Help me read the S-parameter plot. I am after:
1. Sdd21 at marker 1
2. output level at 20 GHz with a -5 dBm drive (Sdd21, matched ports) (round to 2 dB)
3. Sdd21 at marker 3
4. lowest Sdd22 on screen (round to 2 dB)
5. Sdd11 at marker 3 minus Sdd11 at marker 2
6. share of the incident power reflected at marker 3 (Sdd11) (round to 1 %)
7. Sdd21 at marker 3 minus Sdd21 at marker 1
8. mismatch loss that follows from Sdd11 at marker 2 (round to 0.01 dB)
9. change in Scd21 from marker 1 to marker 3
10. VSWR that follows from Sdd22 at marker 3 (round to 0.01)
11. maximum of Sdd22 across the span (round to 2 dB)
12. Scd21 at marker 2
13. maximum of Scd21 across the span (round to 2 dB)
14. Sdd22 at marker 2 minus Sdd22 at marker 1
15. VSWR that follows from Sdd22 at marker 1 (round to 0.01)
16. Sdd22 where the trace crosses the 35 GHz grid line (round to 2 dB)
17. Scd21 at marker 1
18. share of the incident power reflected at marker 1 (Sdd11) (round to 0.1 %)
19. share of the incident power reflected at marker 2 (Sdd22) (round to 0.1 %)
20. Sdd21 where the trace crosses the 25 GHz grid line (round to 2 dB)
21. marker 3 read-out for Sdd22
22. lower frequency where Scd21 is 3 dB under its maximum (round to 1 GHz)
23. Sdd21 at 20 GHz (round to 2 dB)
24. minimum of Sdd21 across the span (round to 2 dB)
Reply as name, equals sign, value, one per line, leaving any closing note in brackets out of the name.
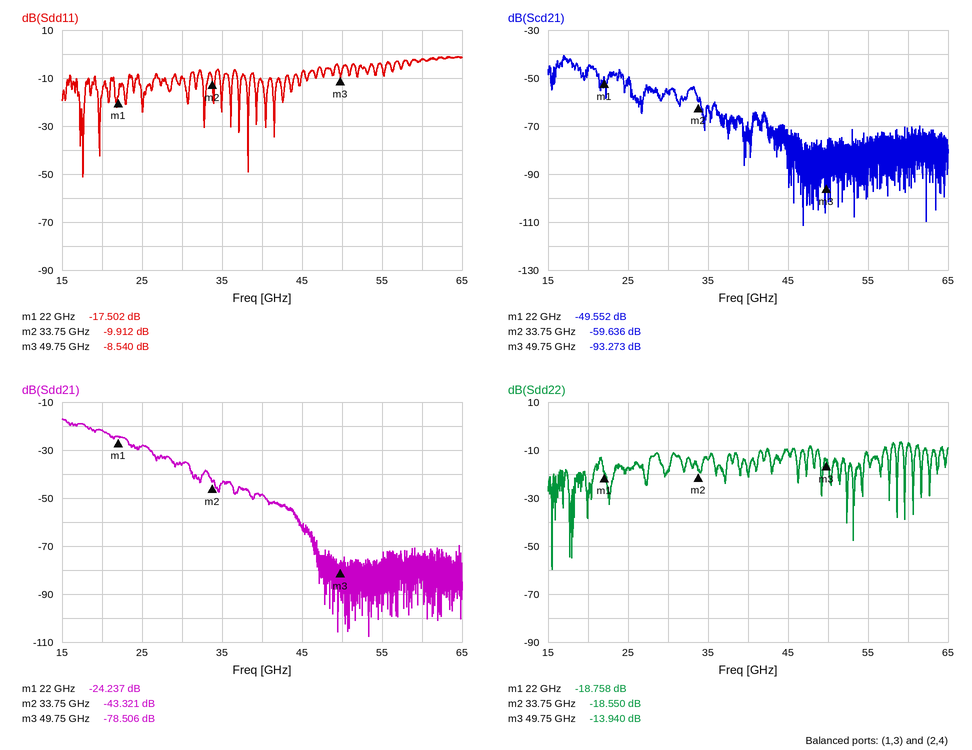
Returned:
Sdd21 at marker 1 = -24.237 dB
output level at 20 GHz with a -5 dBm drive (Sdd21, matched ports) = -26 dBm
Sdd21 at marker 3 = -78.506 dB
lowest Sdd22 on screen = -60 dB
Sdd11 at marker 3 minus Sdd11 at marker 2 = 1.372 dB
share of the incident power reflected at marker 3 (Sdd11) = 14 %
Sdd21 at marker 3 minus Sdd21 at marker 1 = -54.269 dB
mismatch loss that follows from Sdd11 at marker 2 = 0.47 dB
change in Scd21 from marker 1 to marker 3 = -43.721 dB
VSWR that follows from Sdd22 at marker 3 = 1.50
maximum of Sdd22 across the span = -6 dB
Scd21 at marker 2 = -59.636 dB
maximum of Scd21 across the span = -40 dB
Sdd22 at marker 2 minus Sdd22 at marker 1 = 0.208 dB
VSWR that follows from Sdd22 at marker 1 = 1.26
Sdd22 where the trace crosses the 35 GHz grid line = -14 dB
Scd21 at marker 1 = -49.552 dB
share of the incident power reflected at marker 1 (Sdd11) = 1.8 %
share of the incident power reflected at marker 2 (Sdd22) = 1.4 %
Sdd21 where the trace crosses the 25 GHz grid line = -28 dB
marker 3 read-out for Sdd22 = -13.940 dB
lower frequency where Scd21 is 3 dB under its maximum = 17 GHz
Sdd21 at 20 GHz = -22 dB
minimum of Sdd21 across the span = -108 dB
